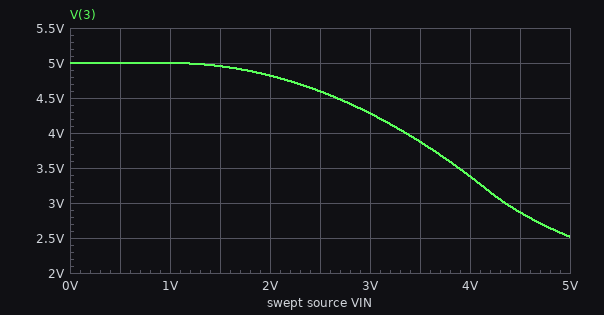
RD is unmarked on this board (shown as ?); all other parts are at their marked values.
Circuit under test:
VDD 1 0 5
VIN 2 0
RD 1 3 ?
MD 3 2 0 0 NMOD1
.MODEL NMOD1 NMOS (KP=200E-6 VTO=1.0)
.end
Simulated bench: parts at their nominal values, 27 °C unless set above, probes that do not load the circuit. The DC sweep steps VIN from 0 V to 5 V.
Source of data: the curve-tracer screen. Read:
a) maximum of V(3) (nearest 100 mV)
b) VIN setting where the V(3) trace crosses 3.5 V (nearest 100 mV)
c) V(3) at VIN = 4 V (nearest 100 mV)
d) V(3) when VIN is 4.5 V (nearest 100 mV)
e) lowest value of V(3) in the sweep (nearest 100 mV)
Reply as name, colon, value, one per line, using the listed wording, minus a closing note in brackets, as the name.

maximum of V(3): 5.0 V
VIN setting where the V(3) trace crosses 3.5 V: 3.9 V
V(3) at VIN = 4 V: 3.4 V
V(3) when VIN is 4.5 V: 2.9 V
lowest value of V(3) in the sweep: 2.5 V
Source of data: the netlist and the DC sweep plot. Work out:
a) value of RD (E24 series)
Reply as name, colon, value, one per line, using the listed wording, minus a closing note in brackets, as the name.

value of RD: 1.8 kΩ
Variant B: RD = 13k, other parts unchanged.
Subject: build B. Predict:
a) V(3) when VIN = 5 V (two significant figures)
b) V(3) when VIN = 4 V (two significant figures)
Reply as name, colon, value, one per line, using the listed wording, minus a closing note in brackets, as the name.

V(3) when VIN = 5 V: 460 mV
V(3) when VIN = 4 V: 630 mV
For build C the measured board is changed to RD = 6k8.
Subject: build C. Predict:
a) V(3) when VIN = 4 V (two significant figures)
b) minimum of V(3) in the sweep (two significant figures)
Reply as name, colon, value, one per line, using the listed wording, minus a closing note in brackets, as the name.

V(3) when VIN = 4 V: 1.2 V
minimum of V(3) in the sweep: 850 mV
